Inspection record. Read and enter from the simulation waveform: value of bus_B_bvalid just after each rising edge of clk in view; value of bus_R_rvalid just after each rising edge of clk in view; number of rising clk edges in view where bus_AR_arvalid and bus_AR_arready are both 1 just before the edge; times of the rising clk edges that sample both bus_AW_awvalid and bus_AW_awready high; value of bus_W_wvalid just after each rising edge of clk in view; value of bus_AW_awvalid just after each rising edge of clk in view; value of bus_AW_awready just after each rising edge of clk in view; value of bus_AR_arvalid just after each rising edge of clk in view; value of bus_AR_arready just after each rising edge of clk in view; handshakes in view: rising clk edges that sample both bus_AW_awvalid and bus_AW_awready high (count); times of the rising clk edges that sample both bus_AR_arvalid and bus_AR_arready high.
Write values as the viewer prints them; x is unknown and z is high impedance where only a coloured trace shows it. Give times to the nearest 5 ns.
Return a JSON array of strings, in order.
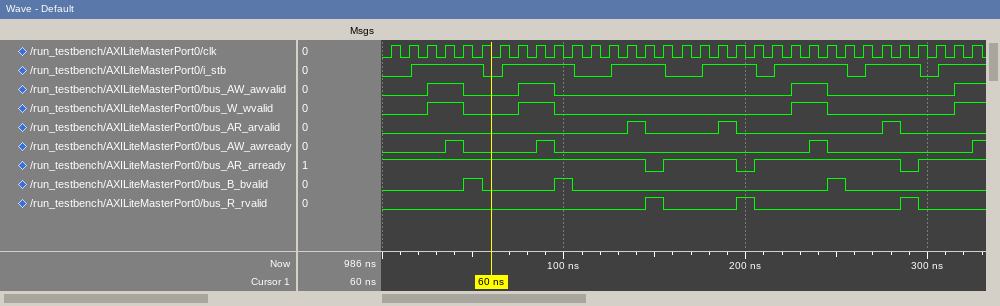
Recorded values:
["0 0 0 0 1 0 0 0 0 1 0 0 0 0 0 0 0 0 0 0 0 0 0 0 1 0 0 0 0 0 0 0 0", "0 0 0 0 0 0 0 0 0 0 0 0 0 0 1 0 0 0 0 1 0 0 0 0 0 0 0 0 1 0 0 0 0", "3", "45 ns, 95 ns, 245 ns", "0 0 1 1 0 0 0 1 1 0 0 0 0 0 0 0 0 0 0 0 0 0 1 1 0 0 0 0 0 0 0 1 1", "0 0 1 1 0 0 0 1 1 0 0 0 0 0 0 0 0 0 0 0 0 0 1 1 0 0 0 0 0 0 0 1 1", "0 0 0 1 0 0 0 0 1 0 0 0 0 0 0 0 0 0 0 0 0 0 0 1 0 0 0 0 0 0 0 0 1", "0 0 0 0 0 0 0 0 0 0 0 0 0 1 0 0 0 0 1 0 0 0 0 0 0 0 0 1 0 0 0 0 0", "1 1 1 1 1 1 1 1 1 1 1 1 1 1 0 1 1 1 1 0 1 1 1 1 1 1 1 1 0 1 1 1 1", "3", "145 ns, 195 ns, 285 ns"]
